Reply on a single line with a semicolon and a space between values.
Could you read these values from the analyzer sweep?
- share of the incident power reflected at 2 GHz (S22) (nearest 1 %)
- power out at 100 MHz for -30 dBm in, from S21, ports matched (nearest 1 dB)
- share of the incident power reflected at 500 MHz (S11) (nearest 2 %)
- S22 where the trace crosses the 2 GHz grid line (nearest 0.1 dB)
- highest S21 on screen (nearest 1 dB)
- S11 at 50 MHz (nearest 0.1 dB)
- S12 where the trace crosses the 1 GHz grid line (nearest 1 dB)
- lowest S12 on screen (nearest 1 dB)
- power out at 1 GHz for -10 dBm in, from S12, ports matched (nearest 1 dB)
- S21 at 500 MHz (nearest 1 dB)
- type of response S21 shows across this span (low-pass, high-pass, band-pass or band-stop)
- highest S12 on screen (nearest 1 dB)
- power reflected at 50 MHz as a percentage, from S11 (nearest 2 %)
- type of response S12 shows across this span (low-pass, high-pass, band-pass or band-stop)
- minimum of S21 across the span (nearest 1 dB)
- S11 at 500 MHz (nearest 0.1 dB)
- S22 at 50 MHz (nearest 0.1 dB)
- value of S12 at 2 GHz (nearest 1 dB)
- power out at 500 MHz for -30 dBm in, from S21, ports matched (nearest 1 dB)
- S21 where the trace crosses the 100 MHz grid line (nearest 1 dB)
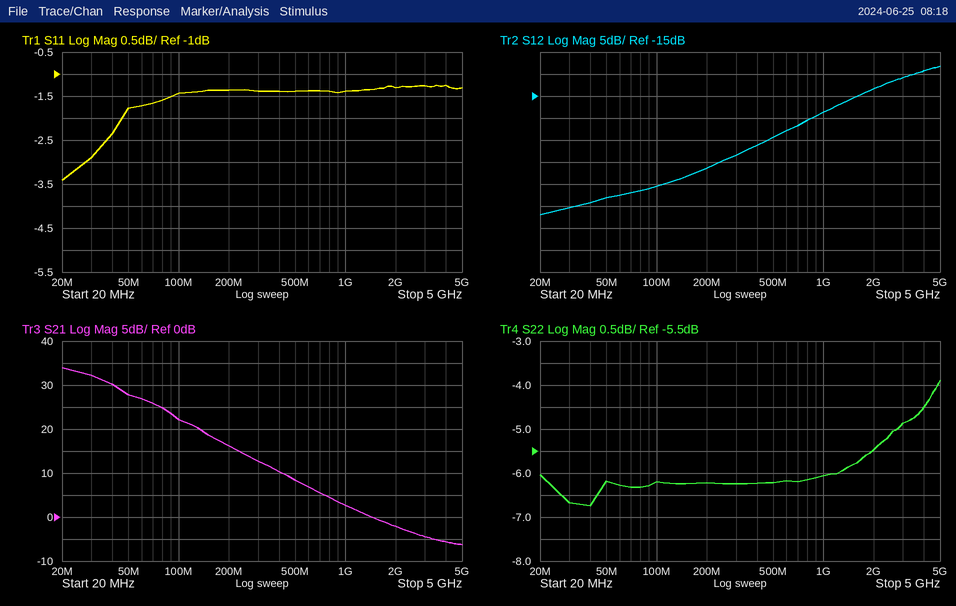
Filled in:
28 %; -8 dBm; 72 %; -5.5 dB; 34 dB; -1.8 dB; -19 dB; -42 dB; -29 dBm; 8 dB; low-pass; -8 dB; 66 %; high-pass; -6 dB; -1.4 dB; -6.2 dB; -13 dB; -22 dBm; 22 dB
